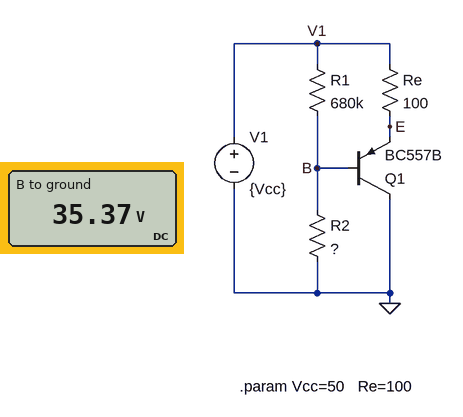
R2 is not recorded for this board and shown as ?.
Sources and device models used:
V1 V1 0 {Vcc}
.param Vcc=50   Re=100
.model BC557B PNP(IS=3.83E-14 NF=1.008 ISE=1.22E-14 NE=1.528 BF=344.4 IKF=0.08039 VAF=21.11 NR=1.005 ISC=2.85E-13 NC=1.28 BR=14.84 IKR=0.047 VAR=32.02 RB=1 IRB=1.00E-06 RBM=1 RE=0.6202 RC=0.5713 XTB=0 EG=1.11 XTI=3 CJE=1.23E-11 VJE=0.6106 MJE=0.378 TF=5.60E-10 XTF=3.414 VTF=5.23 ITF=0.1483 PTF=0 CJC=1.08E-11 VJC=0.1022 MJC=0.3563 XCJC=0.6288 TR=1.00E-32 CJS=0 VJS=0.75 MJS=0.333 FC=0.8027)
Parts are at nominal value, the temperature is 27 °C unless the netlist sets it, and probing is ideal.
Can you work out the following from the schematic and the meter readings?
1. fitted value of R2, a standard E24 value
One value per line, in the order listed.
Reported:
130 kΩ
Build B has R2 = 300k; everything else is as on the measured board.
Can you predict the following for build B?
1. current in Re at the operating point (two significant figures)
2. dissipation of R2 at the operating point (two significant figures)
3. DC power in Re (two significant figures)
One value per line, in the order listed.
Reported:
87 mA
5.5 mW
760 mW
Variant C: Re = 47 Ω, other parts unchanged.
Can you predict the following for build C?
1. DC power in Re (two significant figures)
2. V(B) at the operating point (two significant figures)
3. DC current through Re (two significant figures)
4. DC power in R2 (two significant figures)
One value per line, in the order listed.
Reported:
1.4 W
41 V
170 mA
13 mW
